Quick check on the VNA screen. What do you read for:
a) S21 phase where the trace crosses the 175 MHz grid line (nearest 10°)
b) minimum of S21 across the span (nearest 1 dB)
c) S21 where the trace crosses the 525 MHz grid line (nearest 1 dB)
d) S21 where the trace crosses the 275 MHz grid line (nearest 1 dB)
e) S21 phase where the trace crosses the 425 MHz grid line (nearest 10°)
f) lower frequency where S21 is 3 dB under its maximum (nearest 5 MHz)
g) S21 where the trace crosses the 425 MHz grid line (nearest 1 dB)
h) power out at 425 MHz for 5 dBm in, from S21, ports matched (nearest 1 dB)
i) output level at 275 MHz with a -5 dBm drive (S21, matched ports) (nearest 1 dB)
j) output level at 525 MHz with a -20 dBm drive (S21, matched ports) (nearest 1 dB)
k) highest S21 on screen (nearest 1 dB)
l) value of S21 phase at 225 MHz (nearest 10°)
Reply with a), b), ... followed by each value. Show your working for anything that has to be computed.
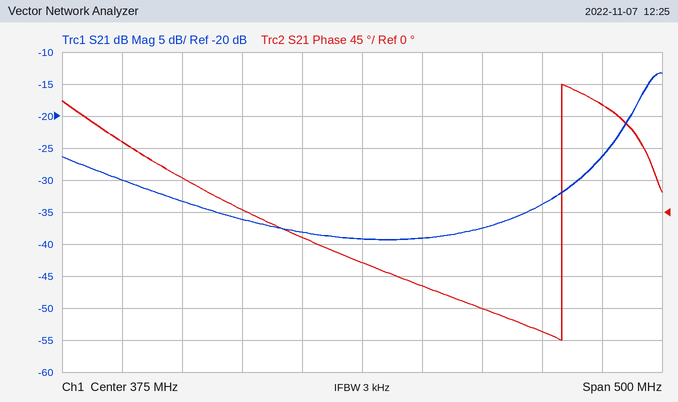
a) 100°
b) -39 dB
c) -34 dB
d) -36 dB
e) -100°
f) 610 MHz
g) -39 dB
h) 5 dBm + (-39 dB) = -34 dBm
i) -5 dBm + (-36 dB) = -41 dBm
j) -20 dBm + (-34 dB) = -54 dBm
k) -13 dB
l) 50°
